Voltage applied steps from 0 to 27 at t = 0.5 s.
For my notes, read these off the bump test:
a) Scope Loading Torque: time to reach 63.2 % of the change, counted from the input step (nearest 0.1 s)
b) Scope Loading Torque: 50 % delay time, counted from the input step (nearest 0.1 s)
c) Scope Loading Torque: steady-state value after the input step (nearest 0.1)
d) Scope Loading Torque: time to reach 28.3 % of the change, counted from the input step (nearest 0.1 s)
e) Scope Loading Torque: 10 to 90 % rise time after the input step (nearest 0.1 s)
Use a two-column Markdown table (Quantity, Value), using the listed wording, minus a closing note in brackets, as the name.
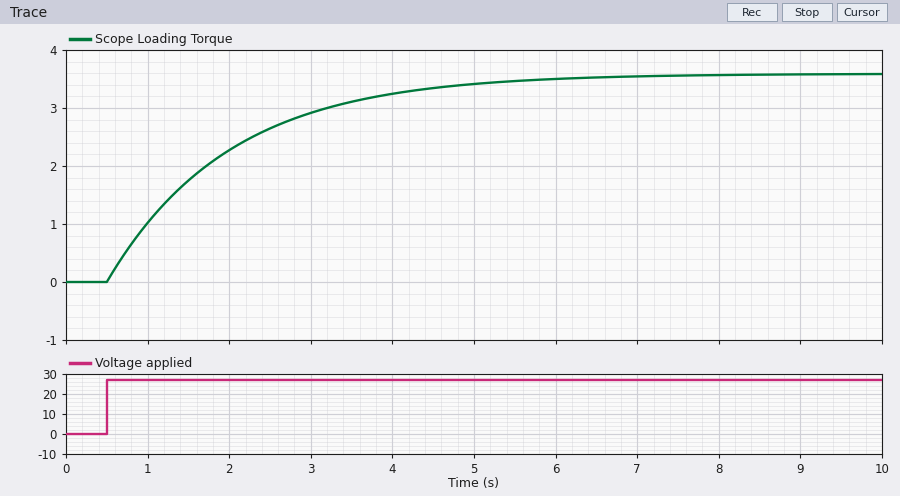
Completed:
| Quantity | Value |
|---|---|
| Scope Loading Torque: time to reach 63.2 % of the change, counted from the input step | 1.5 s |
| Scope Loading Torque: 50 % delay time, counted from the input step | 1.0 s |
| Scope Loading Torque: steady-state value after the input step | 3.6 |
| Scope Loading Torque: time to reach 28.3 % of the change, counted from the input step | 0.5 s |
| Scope Loading Torque: 10 to 90 % rise time after the input step | 3.3 s |
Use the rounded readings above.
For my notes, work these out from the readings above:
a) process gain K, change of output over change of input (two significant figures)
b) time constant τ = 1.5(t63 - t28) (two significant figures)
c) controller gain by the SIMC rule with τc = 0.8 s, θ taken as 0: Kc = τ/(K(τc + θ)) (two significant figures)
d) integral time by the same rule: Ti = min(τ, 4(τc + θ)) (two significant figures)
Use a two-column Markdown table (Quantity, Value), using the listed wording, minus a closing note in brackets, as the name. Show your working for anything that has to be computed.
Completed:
| Quantity | Value |
|---|---|
| process gain K, change of output over change of input | (3.6 - 0) / 27 = 0.13 |
| time constant τ = 1.5(t63 - t28) | 1.5 × (1.5 - 0.5) = 1.5 s |
| controller gain by the SIMC rule with τc = 0.8 s, θ taken as 0: Kc = τ/(K(τc + θ)) | 1.5 / (0.13 × (0.8 + 0)) = 14 |
| integral time by the same rule: Ti = min(τ, 4(τc + θ)) | min(1.5, 4 × (0.8 + 0)) = 1.5 s |
